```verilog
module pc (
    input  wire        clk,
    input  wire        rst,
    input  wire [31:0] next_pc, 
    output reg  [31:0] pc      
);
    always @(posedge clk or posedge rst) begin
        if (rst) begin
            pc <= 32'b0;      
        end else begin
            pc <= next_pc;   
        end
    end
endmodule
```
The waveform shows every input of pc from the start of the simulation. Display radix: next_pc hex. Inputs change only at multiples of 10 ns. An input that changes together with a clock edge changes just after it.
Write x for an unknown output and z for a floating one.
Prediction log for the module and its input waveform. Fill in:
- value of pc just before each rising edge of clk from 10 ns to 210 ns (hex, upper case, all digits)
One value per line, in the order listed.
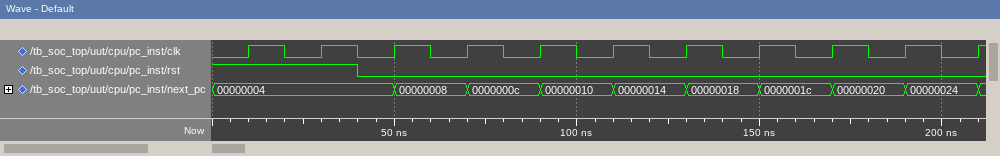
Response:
00000000, 00000000, 00000000, 00000004, 00000008, 0000000C, 00000010, 00000014, 00000018, 0000001C, 00000020
